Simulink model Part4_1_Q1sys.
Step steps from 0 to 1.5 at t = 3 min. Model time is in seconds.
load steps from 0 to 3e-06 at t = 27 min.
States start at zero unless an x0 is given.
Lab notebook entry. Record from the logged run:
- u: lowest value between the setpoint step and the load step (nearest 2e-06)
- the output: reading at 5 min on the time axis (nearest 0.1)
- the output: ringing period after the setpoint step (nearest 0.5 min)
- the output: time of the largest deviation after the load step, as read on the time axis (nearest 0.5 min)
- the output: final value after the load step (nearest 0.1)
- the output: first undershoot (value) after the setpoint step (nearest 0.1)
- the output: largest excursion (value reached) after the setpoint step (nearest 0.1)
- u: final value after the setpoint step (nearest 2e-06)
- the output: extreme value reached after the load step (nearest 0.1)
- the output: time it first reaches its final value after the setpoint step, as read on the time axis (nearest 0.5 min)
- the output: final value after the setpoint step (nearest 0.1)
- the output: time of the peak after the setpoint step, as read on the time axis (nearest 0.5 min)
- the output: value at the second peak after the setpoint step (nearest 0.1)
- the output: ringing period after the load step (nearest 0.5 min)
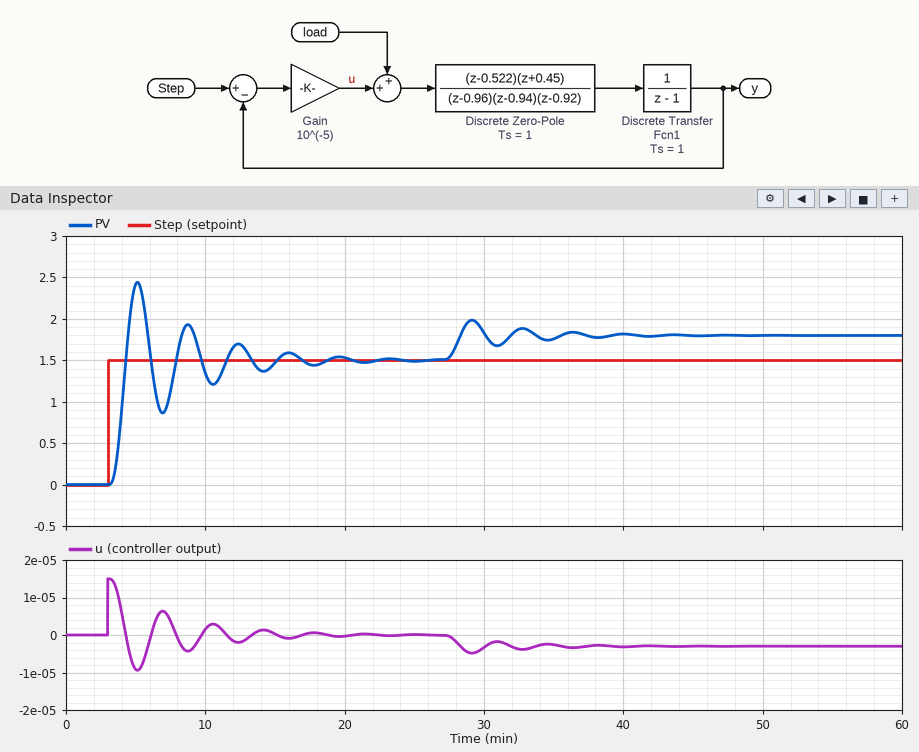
-0.000010
2.4
3.5 min
29.0 min
1.8
0.9
2.4
0.000000
2.0
4.5 min
1.5
5.0 min
1.9
3.5 min
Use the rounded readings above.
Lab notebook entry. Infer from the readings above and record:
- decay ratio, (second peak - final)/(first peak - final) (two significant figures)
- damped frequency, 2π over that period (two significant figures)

0.44
1.8 rad/min
